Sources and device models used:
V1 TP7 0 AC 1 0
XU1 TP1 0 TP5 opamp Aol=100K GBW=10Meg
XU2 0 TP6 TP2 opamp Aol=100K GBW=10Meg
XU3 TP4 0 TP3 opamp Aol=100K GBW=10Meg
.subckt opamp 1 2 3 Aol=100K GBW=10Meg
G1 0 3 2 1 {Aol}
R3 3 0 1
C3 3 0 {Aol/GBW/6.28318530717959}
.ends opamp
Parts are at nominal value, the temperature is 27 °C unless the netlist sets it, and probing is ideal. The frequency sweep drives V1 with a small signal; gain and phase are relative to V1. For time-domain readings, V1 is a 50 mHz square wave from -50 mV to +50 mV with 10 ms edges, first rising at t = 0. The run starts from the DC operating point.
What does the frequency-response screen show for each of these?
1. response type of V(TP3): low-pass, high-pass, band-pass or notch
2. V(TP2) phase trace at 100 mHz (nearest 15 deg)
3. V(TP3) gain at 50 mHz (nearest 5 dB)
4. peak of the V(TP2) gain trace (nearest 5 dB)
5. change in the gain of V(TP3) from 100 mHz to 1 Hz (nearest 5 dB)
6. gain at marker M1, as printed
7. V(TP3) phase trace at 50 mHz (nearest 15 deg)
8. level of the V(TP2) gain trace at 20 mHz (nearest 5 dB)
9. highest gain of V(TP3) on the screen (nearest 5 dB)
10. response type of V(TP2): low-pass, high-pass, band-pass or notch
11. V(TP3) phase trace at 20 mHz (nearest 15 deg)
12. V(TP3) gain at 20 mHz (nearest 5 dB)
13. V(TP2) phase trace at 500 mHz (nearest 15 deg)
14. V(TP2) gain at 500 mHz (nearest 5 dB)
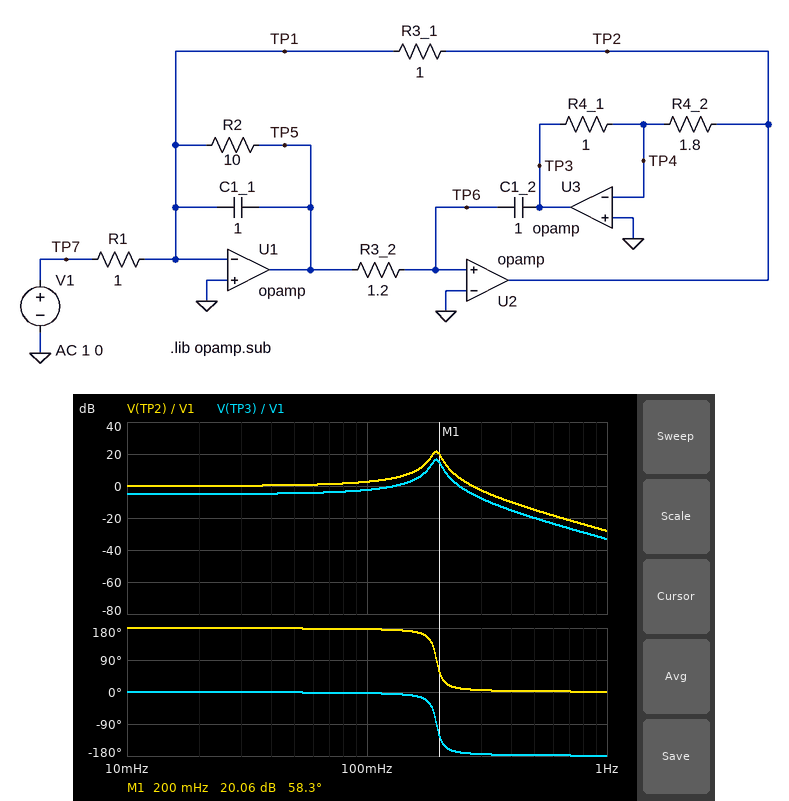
low-pass
180 deg
-5 dB
20 dB
-30 dB
20.06 dB
0 deg
0 dB
15 dB
low-pass
0 deg
-5 dB
0 deg
-15 dB
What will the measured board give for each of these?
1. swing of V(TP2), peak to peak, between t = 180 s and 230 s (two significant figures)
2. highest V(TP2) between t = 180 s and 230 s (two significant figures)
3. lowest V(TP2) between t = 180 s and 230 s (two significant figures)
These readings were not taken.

210 mV
110 mV
-110 mV
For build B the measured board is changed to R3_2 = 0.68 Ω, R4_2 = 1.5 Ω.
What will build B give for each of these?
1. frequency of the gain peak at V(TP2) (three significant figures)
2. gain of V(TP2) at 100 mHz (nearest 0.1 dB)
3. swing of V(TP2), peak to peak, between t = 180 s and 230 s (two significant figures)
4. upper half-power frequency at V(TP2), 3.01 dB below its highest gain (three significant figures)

236 mHz
1.7 dB
330 mV
244 mHz
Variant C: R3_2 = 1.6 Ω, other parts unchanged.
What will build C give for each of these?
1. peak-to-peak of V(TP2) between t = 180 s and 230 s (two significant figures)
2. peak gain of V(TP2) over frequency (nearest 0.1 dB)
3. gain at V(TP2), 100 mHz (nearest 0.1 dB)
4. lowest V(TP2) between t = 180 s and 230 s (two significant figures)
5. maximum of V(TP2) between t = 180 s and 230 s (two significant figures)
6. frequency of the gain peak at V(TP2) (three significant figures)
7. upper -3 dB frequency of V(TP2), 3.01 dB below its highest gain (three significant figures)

290 mV
20.5 dB
3.7 dB
-140 mV
140 mV
168 mHz
176 mHz
